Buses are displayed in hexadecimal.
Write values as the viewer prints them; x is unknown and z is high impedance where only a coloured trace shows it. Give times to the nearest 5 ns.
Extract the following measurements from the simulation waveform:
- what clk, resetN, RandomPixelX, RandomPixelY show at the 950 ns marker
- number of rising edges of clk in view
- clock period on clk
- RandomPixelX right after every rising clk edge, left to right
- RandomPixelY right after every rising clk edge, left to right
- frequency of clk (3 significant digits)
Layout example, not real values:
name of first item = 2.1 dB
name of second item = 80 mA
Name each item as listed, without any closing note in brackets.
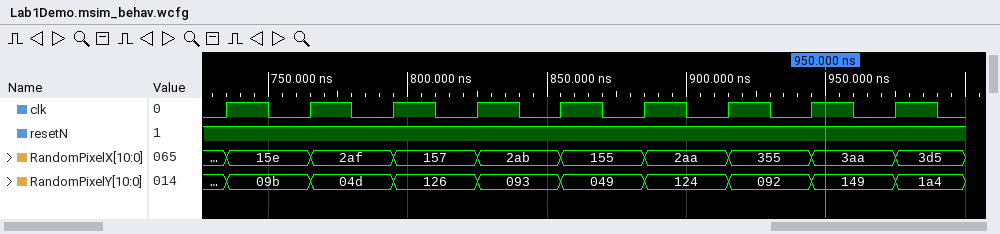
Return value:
what clk, resetN, RandomPixelX, RandomPixelY show at the 950 ns marker = clk=1, resetN=1, RandomPixelX=3aa, RandomPixelY=149
number of rising edges of clk in view = 9
clock period on clk = 30 ns
RandomPixelX right after every rising clk edge, left to right = 15e, 2af, 157, 2ab, 155, 2aa, 355, 3aa, 3d5
RandomPixelY right after every rising clk edge, left to right = 09b, 04d, 126, 093, 049, 124, 092, 149, 1a4
frequency of clk = 33.3 MHz
